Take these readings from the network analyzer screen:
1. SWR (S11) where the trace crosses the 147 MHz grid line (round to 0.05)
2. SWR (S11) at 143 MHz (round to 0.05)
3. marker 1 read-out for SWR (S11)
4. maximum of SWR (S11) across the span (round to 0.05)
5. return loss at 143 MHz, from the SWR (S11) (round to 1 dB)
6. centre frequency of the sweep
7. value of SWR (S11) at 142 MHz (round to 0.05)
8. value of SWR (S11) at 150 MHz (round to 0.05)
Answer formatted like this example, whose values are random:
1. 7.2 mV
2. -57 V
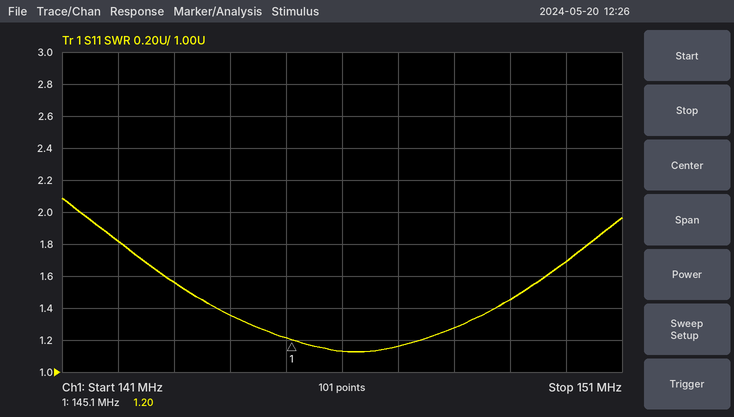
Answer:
1. 1.15
2. 1.55
3. 1.20
4. 2.10
5. 13 dB
6. 146 MHz
7. 1.80
8. 1.70
